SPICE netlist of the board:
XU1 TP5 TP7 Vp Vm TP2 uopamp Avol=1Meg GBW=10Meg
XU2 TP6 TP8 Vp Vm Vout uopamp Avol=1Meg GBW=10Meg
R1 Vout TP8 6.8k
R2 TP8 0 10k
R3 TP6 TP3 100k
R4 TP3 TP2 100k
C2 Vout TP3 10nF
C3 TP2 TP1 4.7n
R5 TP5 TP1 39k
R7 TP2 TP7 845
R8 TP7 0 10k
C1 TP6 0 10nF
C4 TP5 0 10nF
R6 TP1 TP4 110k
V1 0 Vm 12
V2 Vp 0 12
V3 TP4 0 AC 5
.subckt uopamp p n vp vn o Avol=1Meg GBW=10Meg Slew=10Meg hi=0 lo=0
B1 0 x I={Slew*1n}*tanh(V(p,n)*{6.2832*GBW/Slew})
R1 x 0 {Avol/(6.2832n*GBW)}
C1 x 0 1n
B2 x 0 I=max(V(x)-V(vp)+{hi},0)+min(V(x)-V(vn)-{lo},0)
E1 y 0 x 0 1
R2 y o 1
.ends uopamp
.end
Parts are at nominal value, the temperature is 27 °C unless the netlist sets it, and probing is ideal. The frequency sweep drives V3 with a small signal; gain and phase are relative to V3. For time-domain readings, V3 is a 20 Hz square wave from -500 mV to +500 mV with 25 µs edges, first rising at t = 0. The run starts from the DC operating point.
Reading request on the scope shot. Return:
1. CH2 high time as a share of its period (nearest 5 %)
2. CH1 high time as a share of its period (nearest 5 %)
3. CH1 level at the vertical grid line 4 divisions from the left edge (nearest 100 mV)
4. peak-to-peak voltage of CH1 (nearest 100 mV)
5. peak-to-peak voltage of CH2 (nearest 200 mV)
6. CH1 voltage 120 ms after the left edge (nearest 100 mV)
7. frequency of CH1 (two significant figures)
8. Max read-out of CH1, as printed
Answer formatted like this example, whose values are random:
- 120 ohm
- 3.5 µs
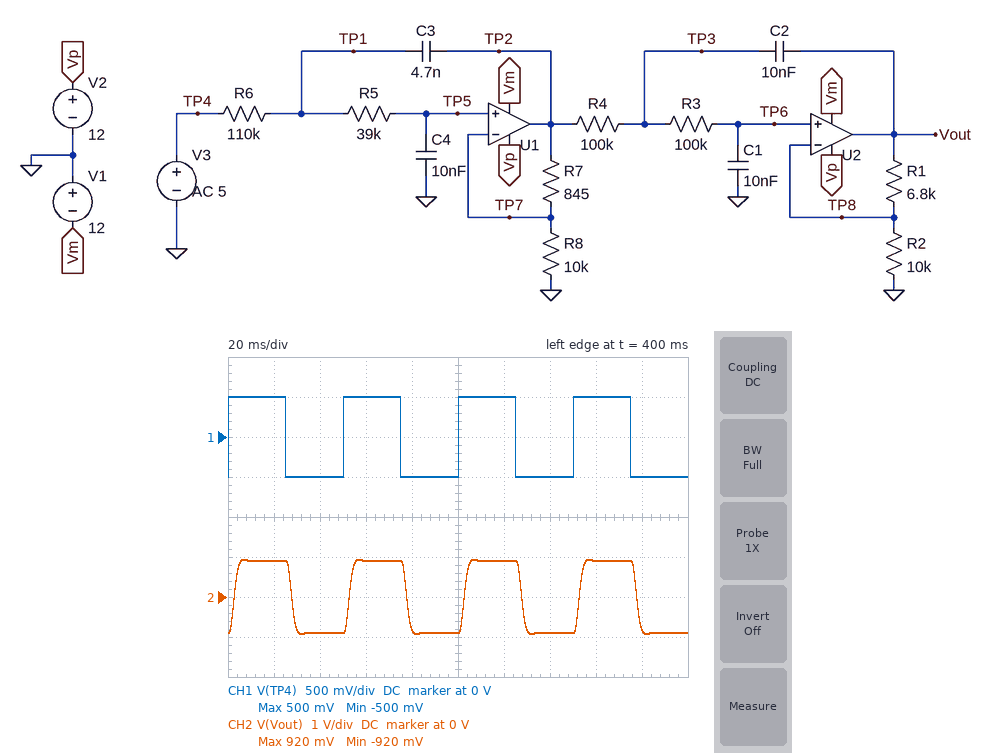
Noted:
- 50 %
- 50 %
- -500 mV
- 1.0 V
- 1.8 V
- 500 mV
- 20 Hz
- 500 mV
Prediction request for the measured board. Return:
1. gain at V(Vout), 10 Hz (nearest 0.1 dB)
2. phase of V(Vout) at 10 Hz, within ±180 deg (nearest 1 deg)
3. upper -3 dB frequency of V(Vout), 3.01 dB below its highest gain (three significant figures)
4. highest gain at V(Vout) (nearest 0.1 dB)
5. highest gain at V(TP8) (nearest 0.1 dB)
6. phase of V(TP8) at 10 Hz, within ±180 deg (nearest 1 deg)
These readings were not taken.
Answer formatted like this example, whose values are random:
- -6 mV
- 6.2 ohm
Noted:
- 5.2 dB
- -10 deg
- 110 Hz
- 5.2 dB
- 0.7 dB
- -10 deg
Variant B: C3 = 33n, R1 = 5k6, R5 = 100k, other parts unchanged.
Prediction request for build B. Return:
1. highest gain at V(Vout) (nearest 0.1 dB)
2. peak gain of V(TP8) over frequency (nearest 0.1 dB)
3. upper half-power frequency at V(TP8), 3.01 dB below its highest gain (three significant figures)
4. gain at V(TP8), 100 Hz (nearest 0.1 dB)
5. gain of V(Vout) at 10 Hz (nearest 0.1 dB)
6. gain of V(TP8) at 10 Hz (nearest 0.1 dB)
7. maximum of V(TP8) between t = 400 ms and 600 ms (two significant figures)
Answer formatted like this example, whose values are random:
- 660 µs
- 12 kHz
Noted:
- 6.0 dB
- 2.2 dB
- 95.1 Hz
- -1.7 dB
- 4.6 dB
- 0.8 dB
- 750 mV
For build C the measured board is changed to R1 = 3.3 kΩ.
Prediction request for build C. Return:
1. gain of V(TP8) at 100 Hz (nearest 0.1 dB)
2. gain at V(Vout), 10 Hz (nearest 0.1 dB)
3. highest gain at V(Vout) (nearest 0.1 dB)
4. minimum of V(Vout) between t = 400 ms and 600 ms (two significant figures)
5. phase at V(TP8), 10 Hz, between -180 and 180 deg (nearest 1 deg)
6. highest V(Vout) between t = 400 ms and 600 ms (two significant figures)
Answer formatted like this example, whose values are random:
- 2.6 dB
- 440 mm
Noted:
- -3.2 dB
- 3.1 dB
- 3.2 dB
- -720 mV
- -11 deg
- 720 mV
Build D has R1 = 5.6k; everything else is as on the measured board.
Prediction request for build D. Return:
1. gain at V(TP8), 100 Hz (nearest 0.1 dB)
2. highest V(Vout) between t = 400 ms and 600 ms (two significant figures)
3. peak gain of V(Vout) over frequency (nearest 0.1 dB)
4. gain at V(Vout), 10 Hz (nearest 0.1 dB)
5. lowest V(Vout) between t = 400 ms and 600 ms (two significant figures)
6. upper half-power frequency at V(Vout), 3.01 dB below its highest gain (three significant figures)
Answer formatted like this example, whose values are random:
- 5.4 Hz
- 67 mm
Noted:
- -2.3 dB
- 850 mV
- 4.6 dB
- 4.5 dB
- -850 mV
- 101 Hz
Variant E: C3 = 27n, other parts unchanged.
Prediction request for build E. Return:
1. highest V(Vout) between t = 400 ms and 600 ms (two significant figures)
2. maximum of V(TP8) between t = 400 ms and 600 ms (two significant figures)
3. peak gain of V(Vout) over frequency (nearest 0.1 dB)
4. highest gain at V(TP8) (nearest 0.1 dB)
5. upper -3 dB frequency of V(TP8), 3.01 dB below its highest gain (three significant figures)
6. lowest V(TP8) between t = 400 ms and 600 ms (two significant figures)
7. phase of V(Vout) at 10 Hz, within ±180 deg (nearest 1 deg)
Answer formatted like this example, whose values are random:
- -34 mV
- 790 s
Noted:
- 1.2 V
- 690 mV
- 5.7 dB
- 1.2 dB
- 142 Hz
- -690 mV
- -9 deg
